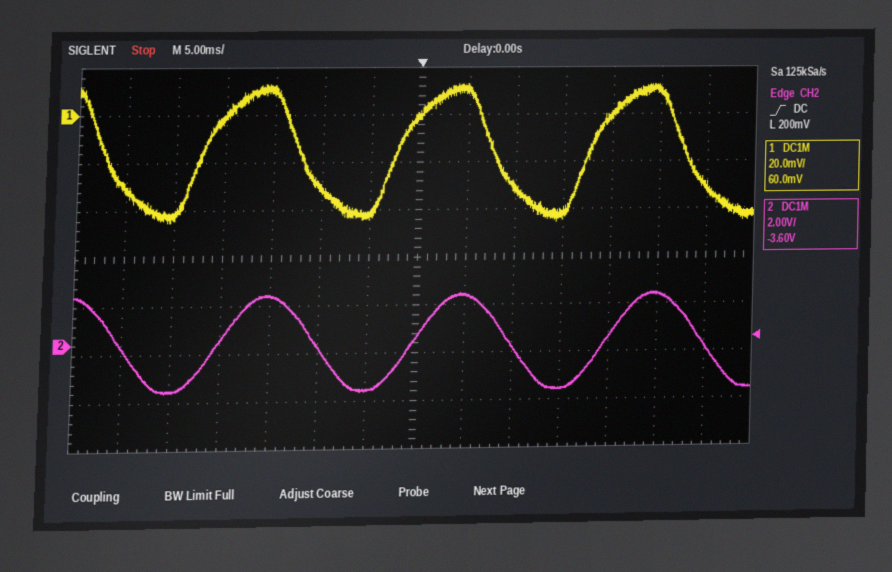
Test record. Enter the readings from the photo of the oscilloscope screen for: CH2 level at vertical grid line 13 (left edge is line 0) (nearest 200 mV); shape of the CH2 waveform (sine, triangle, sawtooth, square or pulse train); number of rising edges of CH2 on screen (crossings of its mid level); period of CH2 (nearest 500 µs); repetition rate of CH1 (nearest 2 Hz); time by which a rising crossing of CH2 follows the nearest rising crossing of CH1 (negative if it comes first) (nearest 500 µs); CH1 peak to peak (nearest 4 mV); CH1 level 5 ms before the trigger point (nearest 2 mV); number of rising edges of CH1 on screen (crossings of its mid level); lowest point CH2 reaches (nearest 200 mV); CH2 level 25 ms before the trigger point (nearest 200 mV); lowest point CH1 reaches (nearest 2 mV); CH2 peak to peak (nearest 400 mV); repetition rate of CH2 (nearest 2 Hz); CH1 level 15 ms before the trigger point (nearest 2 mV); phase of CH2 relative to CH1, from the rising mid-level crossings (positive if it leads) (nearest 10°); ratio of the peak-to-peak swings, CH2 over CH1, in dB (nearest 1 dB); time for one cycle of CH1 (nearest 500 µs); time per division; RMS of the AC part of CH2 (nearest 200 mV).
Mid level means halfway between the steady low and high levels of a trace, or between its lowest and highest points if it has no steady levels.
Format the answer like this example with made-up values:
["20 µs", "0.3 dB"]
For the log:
["-200 mV", "sine", "3", "20.0 ms", "50 Hz", "+2.0 ms", "56 mV", "-42 mV", "3", "-2.0 V", "-2.0 V", "-44 mV", "4.0 V", "50 Hz", "10 mV", "-40°", "37 dB", "20.0 ms", "5 ms", "1.4 V"]
